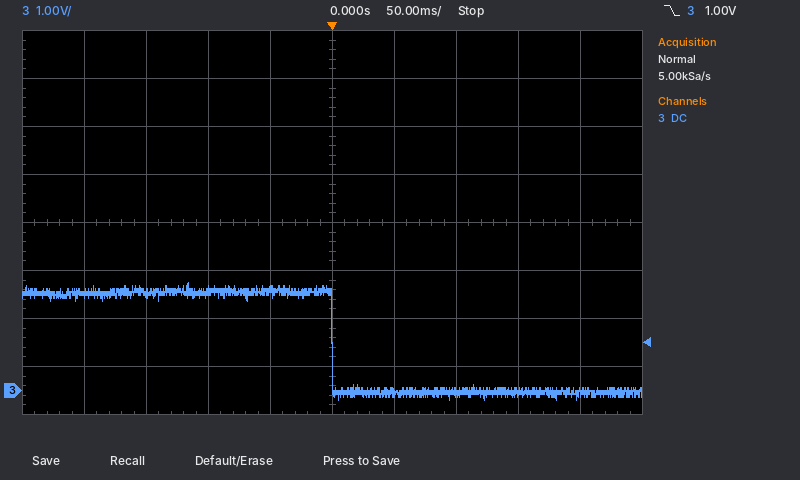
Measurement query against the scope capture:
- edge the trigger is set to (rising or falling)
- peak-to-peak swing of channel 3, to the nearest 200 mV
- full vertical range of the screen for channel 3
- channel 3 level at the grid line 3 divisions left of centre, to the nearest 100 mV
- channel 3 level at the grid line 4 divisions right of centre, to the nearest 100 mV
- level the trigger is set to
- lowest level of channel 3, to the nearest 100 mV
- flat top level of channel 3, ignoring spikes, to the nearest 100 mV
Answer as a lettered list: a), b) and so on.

a) falling
b) 2.4 V
c) 8 V
d) 2.0 V
e) 0.0 V
f) 1.00 V
g) -200 mV
h) 2.1 V
